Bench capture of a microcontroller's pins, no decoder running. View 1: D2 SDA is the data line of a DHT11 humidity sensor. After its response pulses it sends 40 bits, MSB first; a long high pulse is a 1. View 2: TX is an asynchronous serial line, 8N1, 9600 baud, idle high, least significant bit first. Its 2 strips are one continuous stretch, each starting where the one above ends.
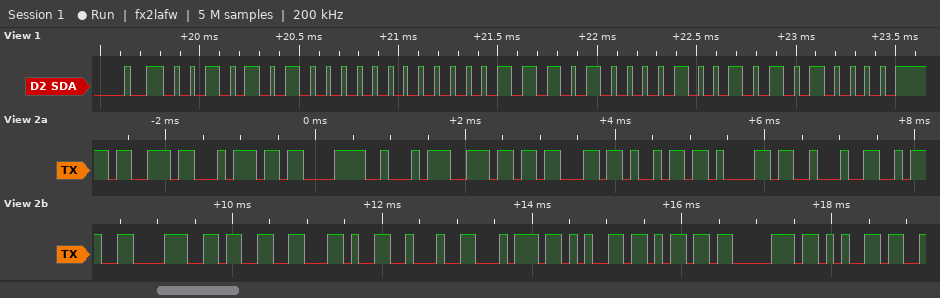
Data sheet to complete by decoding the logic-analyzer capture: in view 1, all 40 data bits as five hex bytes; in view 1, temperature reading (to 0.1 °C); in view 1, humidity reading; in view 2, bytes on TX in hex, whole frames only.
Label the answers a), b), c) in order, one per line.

a) 2A 00 1D 09 50
b) 29.9 °C
c) 42 %
d) 0x73 0x74 0xC3 0xA2 0x6E 0x63 0x69 0x61 0x22 0x3A 0x38 0x33 0x2C 0x22 0x74 0x65 0x6D 0x70 0x65
